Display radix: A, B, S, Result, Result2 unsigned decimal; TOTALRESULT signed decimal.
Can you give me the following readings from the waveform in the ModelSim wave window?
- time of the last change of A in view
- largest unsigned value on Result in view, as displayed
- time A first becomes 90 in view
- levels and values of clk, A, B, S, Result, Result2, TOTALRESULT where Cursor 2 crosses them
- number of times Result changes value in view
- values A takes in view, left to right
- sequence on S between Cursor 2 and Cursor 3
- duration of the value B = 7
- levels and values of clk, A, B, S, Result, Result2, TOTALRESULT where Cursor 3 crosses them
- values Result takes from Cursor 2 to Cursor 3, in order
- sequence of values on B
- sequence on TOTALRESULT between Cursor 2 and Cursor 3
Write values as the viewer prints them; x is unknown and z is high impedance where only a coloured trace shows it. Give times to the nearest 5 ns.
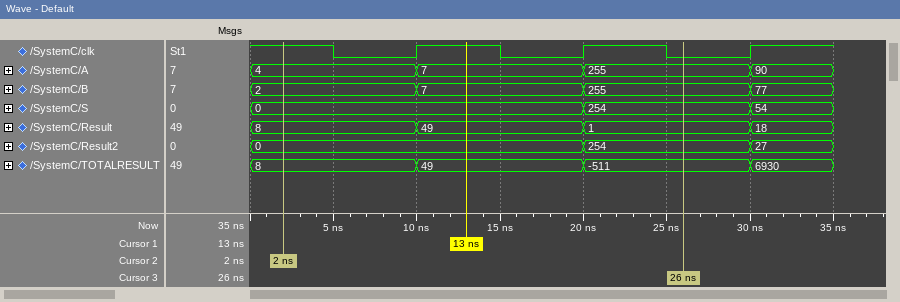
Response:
30 ns
49
30 ns
clk=1, A=4, B=2, S=0, Result=8, Result2=0, TOTALRESULT=8
3
4, 7, 255, 90
0, 254
10 ns
clk=0, A=255, B=255, S=254, Result=1, Result2=254, TOTALRESULT=-511
8, 49, 1
2, 7, 255, 77
8, 49, -511
